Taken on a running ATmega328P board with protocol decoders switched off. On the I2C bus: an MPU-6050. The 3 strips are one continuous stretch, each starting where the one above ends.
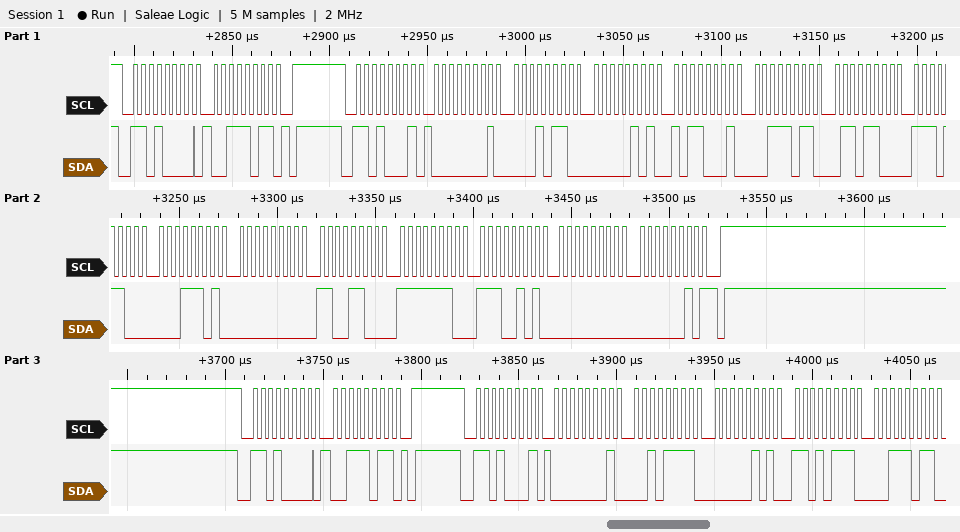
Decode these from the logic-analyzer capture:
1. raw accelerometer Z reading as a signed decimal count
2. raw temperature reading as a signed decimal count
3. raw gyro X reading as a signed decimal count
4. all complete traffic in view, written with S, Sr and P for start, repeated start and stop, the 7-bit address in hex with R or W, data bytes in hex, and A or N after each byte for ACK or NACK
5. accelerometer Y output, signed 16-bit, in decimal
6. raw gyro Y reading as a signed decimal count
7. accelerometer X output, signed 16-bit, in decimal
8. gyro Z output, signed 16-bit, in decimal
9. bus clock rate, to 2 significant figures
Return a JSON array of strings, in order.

["15212", "-5091", "204", "S 68W A 3B A P S 68R A 01 A 16 A 05 A B1 A 3B A 6C A EC A 1D A 00 A CC A FE A E5 A 00 A 02 N P S 68W A 3B A P S 68R A 01 A 2F A 05 A D7 A 3B A", "1457", "-283", "278", "2", "250 kHz"]
